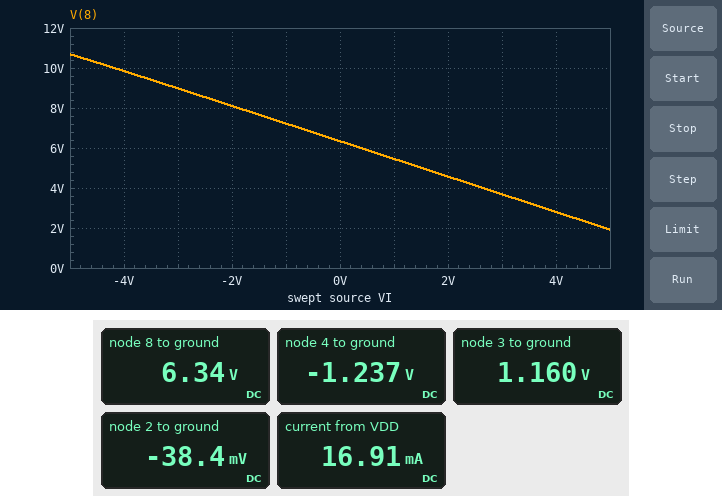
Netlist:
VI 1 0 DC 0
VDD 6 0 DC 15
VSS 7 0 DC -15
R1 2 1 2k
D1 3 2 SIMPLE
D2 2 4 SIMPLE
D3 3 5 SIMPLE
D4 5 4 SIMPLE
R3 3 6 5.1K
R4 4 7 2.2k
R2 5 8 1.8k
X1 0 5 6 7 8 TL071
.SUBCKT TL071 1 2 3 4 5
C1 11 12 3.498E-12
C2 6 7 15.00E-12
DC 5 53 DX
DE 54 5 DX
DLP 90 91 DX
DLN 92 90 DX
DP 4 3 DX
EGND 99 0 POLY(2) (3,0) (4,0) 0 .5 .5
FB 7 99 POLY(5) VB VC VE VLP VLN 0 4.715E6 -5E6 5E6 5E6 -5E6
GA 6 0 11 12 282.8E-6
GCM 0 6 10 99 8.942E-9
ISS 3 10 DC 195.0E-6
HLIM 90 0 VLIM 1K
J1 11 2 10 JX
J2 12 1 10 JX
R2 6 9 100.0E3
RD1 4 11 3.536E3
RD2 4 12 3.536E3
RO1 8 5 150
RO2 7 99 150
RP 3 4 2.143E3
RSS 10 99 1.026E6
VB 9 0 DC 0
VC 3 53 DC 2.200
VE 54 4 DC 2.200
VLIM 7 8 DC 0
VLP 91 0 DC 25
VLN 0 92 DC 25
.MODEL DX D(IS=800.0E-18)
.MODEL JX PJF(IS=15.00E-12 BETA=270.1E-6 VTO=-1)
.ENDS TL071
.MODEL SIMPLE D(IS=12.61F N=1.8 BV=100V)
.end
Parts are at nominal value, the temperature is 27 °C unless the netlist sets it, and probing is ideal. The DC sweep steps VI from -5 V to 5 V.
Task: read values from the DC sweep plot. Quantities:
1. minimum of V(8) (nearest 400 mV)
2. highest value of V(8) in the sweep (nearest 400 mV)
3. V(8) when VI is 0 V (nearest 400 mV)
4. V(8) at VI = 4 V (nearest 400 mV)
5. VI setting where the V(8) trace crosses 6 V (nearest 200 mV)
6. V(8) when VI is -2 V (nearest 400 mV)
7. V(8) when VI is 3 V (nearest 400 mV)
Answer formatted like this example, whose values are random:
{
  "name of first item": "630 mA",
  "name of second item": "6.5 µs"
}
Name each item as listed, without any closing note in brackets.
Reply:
{
  "minimum of V(8)": "2.0 V",
  "highest value of V(8) in the sweep": "10.8 V",
  "V(8) when VI is 0 V": "6.4 V",
  "V(8) at VI = 4 V": "2.8 V",
  "VI setting where the V(8) trace crosses 6 V": "400 mV",
  "V(8) when VI is -2 V": "8.0 V",
  "V(8) when VI is 3 V": "3.6 V"
}
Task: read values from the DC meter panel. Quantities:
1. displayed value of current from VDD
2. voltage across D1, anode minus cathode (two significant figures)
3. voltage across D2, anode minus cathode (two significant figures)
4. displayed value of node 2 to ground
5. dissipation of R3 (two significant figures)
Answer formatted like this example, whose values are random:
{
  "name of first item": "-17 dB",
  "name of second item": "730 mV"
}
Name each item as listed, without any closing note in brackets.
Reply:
{
  "displayed value of current from VDD": "16.91 mA",
  "voltage across D1, anode minus cathode": "1.2 V",
  "voltage across D2, anode minus cathode": "1.2 V",
  "displayed value of node 2 to ground": "-38.4 mV",
  "dissipation of R3": "38 mW"
}
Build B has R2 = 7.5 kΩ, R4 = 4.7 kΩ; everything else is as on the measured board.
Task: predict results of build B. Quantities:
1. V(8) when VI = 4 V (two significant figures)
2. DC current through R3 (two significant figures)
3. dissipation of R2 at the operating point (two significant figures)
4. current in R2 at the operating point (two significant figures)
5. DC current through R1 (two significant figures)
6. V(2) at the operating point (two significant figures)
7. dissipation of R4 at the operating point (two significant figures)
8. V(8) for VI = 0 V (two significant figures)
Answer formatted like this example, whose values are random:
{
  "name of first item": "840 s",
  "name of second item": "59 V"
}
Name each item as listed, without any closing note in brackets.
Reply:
{
  "V(8) when VI = 4 V": "-13 V",
  "DC current through R3": "2.7 mA",
  "dissipation of R2 at the operating point": "390 µW",
  "current in R2 at the operating point": "230 µA",
  "DC current through R1": "1.9 µA",
  "V(2) at the operating point": "-3.7 mV",
  "dissipation of R4 at the operating point": "41 mW",
  "V(8) for VI = 0 V": "1.7 V"
}
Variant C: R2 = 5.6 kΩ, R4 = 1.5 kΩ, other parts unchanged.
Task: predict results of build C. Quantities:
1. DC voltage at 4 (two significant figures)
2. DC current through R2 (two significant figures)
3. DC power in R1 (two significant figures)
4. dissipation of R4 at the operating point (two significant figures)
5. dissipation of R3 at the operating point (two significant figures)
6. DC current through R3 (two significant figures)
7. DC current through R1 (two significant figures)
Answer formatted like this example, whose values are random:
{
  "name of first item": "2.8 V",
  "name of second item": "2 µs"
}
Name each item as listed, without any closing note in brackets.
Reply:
{
  "DC voltage at 4": "-3.9 V",
  "DC current through R2": "2.9 mA",
  "DC power in R1": "3.5 mW",
  "dissipation of R4 at the operating point": "83 mW",
  "dissipation of R3 at the operating point": "53 mW",
  "DC current through R3": "3.2 mA",
  "DC current through R1": "1.3 mA"
}
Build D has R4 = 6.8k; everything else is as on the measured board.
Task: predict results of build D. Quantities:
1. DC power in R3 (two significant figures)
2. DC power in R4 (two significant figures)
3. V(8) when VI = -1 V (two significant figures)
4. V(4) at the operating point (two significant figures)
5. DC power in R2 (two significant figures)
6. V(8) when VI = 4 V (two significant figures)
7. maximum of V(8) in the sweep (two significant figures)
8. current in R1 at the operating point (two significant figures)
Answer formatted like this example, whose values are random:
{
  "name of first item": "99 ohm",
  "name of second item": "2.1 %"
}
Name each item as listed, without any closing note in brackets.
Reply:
{
  "DC power in R3": "37 mW",
  "DC power in R4": "28 mW",
  "V(8) when VI = -1 V": "-320 mV",
  "V(4) at the operating point": "-1.2 V",
  "DC power in R2": "800 µW",
  "V(8) when VI = 4 V": "-4.6 V",
  "maximum of V(8) in the sweep": "3.1 V",
  "current in R1 at the operating point": "6.5 µA"
}
